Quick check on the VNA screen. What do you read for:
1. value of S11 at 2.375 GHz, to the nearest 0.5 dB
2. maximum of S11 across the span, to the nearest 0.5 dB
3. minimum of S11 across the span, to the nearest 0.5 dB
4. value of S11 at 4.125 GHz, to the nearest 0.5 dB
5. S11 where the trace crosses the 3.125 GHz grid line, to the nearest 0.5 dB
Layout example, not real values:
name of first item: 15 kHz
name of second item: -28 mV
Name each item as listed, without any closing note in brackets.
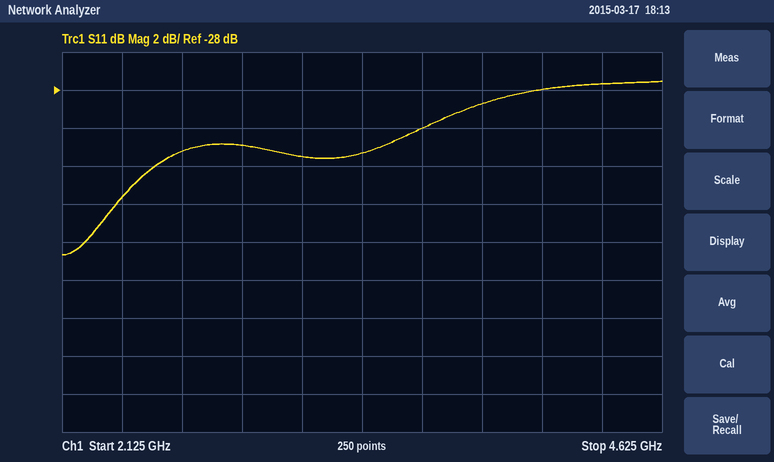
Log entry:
value of S11 at 2.375 GHz, to the nearest 0.5 dB: -33.5 dB
maximum of S11 across the span, to the nearest 0.5 dB: -27.5 dB
minimum of S11 across the span, to the nearest 0.5 dB: -36.5 dB
value of S11 at 4.125 GHz, to the nearest 0.5 dB: -28.0 dB
S11 where the trace crosses the 3.125 GHz grid line, to the nearest 0.5 dB: -31.5 dB
